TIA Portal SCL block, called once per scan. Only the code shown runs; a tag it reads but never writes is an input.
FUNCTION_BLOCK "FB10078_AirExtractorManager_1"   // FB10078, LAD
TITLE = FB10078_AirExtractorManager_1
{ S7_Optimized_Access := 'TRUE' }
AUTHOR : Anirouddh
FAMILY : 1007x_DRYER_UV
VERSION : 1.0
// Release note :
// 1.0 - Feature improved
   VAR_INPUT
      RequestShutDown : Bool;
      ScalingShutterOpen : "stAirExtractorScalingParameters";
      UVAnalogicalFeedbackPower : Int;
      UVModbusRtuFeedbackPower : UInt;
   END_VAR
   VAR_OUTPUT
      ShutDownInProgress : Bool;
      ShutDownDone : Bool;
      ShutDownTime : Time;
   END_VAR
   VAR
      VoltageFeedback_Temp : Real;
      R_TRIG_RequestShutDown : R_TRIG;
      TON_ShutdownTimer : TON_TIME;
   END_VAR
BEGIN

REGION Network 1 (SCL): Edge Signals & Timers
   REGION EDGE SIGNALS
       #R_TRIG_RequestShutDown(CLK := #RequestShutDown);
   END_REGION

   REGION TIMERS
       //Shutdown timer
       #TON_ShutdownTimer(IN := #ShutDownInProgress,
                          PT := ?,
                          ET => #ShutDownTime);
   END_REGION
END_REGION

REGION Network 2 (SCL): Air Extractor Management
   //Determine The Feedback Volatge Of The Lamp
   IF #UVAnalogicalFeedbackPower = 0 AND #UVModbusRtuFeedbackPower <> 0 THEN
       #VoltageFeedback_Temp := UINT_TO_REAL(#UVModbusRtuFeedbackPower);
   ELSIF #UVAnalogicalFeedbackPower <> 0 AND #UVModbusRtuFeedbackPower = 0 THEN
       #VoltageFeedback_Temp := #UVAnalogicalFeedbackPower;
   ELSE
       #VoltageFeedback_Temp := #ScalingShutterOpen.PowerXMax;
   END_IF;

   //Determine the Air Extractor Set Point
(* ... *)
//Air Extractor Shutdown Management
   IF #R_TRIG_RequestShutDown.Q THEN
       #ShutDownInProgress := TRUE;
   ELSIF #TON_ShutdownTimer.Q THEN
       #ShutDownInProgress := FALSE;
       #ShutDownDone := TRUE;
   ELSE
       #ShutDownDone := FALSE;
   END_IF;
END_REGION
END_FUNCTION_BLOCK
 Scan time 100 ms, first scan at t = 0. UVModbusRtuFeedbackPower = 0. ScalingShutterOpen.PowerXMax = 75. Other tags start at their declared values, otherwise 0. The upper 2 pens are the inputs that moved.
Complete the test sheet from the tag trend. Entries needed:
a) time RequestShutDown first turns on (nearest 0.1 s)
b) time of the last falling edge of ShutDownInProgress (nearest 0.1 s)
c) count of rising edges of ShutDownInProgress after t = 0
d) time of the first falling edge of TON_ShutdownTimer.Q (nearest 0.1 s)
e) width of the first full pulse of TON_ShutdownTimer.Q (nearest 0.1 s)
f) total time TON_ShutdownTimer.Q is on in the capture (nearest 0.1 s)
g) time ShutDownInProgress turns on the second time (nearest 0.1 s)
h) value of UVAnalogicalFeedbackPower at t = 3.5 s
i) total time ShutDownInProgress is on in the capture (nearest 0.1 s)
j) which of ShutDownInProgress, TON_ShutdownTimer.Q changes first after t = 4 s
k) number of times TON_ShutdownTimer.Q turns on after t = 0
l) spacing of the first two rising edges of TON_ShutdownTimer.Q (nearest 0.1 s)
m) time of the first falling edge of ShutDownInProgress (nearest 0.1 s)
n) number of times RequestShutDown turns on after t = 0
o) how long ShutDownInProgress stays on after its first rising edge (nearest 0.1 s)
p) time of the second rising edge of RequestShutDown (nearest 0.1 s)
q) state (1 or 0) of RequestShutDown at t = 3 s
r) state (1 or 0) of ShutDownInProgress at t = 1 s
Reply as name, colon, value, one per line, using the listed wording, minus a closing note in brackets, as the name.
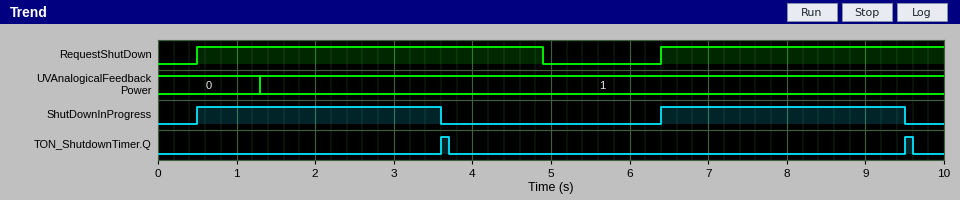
time RequestShutDown first turns on: 0.5 s
time of the last falling edge of ShutDownInProgress: 9.5 s
count of rising edges of ShutDownInProgress after t = 0: 2
time of the first falling edge of TON_ShutdownTimer.Q: 3.7 s
width of the first full pulse of TON_ShutdownTimer.Q: 0.1 s
total time TON_ShutdownTimer.Q is on in the capture: 0.2 s
time ShutDownInProgress turns on the second time: 6.4 s
value of UVAnalogicalFeedbackPower at t = 3.5 s: 1
total time ShutDownInProgress is on in the capture: 6.2 s
which of ShutDownInProgress, TON_ShutdownTimer.Q changes first after t = 4 s: ShutDownInProgress
number of times TON_ShutdownTimer.Q turns on after t = 0: 2
spacing of the first two rising edges of TON_ShutdownTimer.Q: 5.9 s
time of the first falling edge of ShutDownInProgress: 3.6 s
number of times RequestShutDown turns on after t = 0: 2
how long ShutDownInProgress stays on after its first rising edge: 3.1 s
time of the second rising edge of RequestShutDown: 6.4 s
state (1 or 0) of RequestShutDown at t = 3 s: 1
state (1 or 0) of ShutDownInProgress at t = 1 s: 1
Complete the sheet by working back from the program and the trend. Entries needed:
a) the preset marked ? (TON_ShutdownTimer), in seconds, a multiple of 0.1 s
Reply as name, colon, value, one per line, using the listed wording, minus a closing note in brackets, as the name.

the preset marked ? (TON_ShutdownTimer), in seconds, a multiple of 0.1 s: 3.0 s
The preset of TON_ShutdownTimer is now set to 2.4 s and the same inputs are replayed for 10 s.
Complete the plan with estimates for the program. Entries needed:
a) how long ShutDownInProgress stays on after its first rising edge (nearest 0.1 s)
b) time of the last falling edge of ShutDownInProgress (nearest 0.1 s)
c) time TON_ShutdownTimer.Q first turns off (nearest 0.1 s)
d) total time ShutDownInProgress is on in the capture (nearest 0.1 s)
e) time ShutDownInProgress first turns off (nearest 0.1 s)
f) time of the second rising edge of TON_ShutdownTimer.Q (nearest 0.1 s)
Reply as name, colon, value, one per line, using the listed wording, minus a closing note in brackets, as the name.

how long ShutDownInProgress stays on after its first rising edge: 2.5 s
time of the last falling edge of ShutDownInProgress: 8.9 s
time TON_ShutdownTimer.Q first turns off: 3.1 s
total time ShutDownInProgress is on in the capture: 5.0 s
time ShutDownInProgress first turns off: 3.0 s
time of the second rising edge of TON_ShutdownTimer.Q: 8.9 s
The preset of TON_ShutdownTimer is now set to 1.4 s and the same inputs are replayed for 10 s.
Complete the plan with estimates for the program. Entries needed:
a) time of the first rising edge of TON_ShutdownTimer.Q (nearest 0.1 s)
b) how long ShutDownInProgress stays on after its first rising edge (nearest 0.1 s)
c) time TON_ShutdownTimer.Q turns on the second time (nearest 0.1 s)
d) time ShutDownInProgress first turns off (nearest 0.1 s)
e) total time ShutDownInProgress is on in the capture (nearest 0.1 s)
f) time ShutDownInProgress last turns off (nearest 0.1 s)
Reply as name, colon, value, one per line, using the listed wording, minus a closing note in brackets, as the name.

time of the first rising edge of TON_ShutdownTimer.Q: 2.0 s
how long ShutDownInProgress stays on after its first rising edge: 1.5 s
time TON_ShutdownTimer.Q turns on the second time: 7.9 s
time ShutDownInProgress first turns off: 2.0 s
total time ShutDownInProgress is on in the capture: 3.0 s
time ShutDownInProgress last turns off: 7.9 s
